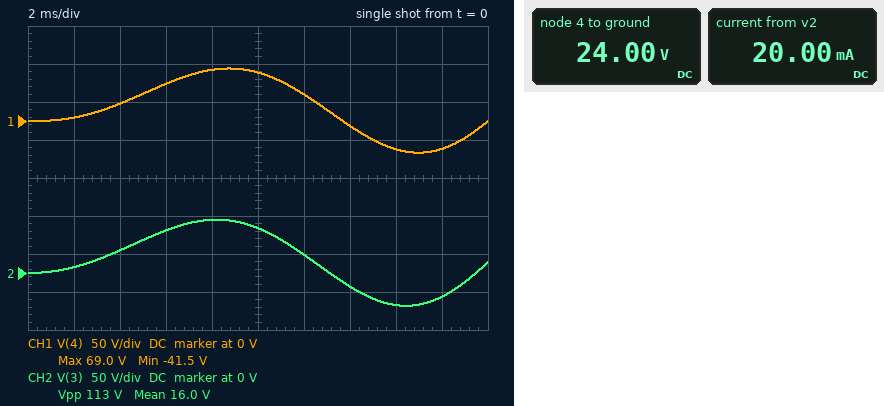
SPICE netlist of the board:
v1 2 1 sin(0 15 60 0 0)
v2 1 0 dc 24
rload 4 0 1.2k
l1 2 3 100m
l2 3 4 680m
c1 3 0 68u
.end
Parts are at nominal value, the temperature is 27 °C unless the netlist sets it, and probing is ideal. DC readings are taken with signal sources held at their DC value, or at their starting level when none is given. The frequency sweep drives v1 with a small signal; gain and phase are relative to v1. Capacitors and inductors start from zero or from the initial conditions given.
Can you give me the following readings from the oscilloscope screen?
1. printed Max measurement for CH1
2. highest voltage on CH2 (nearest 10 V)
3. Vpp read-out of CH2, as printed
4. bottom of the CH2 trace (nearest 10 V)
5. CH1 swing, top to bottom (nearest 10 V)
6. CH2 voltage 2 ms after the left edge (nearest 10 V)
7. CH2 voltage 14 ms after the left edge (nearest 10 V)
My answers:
69.0 V
70 V
113 V
-40 V
110 V
10 V
-20 V
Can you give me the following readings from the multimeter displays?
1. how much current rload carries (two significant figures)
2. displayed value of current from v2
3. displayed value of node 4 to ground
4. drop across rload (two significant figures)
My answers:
20 mA
20.00 mA
24.00 V
24 V
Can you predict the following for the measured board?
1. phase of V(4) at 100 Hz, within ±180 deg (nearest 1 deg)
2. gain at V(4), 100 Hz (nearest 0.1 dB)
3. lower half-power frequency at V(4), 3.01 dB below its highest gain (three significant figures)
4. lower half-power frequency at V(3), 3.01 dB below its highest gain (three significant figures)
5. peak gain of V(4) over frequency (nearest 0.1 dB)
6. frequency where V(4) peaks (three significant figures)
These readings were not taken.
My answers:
162 deg
-5.0 dB
60.3 Hz
60.3 Hz
30.1 dB
61.2 Hz
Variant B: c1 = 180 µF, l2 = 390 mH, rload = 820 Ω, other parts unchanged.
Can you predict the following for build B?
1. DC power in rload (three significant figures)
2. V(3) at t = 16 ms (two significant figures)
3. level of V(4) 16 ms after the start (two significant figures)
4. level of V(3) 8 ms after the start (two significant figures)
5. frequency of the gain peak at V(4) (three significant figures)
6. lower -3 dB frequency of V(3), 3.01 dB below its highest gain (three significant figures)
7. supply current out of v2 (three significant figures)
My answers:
702 mW
36 V
40 V
44 V
37.6 Hz
37.0 Hz
29.3 mA
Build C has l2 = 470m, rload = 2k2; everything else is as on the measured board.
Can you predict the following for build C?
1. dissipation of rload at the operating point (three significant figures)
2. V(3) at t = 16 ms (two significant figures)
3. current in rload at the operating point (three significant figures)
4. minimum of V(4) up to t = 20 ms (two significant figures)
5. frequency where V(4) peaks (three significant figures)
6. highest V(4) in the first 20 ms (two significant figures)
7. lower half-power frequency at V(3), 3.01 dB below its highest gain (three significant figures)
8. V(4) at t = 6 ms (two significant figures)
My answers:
262 mW
-44 V
10.9 mA
-45 V
61.1 Hz
71 V
60.5 Hz
54 V
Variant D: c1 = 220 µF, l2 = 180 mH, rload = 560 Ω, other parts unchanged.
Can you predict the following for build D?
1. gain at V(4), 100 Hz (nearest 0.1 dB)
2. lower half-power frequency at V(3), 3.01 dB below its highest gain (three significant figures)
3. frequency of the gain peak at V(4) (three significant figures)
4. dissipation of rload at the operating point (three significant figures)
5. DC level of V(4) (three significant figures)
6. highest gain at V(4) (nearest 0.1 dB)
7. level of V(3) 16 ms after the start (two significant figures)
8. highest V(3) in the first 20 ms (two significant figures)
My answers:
-17.9 dB
33.3 Hz
34.0 Hz
1.03 W
24.0 V
28.4 dB
44 V
56 V
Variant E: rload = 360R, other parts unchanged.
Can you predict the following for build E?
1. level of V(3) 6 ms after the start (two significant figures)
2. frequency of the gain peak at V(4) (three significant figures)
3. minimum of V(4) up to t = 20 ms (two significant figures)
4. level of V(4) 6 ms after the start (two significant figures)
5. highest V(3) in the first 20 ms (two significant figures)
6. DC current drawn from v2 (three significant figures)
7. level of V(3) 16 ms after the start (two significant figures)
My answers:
55 V
62.6 Hz
-26 V
34 V
68 V
66.7 mA
-37 V
